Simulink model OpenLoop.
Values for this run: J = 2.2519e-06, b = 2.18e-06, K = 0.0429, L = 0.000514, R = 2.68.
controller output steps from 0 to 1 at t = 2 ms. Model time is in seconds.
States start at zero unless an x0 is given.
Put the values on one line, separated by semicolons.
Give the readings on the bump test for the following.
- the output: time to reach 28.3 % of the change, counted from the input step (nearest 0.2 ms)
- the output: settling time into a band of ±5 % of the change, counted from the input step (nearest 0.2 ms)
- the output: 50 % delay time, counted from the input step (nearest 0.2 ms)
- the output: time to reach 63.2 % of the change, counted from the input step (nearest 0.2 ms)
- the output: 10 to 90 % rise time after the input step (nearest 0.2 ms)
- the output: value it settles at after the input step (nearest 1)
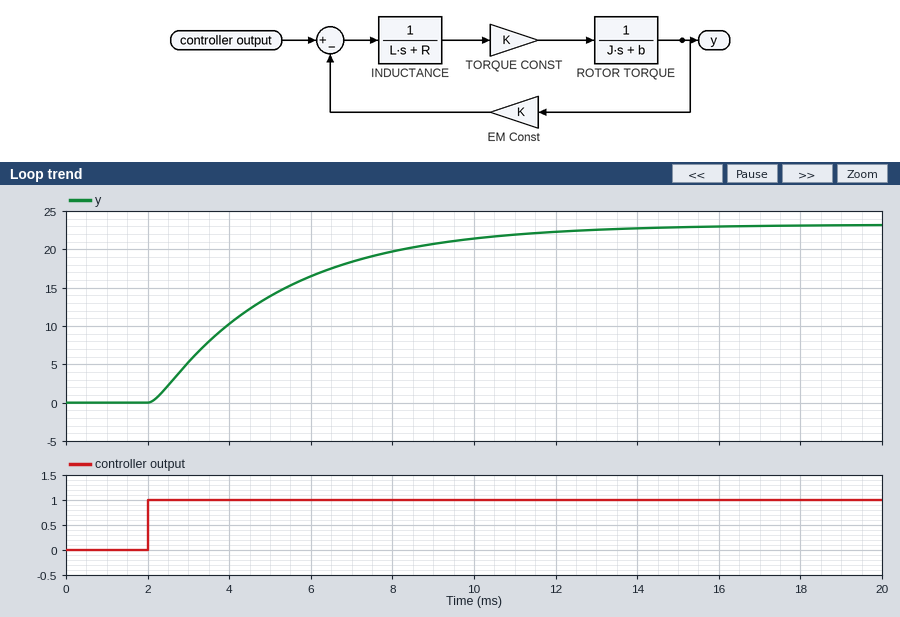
1.2 ms; 9.4 ms; 2.4 ms; 3.2 ms; 6.8 ms; 23
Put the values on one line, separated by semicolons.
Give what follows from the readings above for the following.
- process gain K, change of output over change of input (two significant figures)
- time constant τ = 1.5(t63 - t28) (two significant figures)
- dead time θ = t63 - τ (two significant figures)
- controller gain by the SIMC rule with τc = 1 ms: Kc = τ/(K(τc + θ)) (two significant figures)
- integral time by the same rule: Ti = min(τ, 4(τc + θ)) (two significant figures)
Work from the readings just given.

23; 3.0 ms; 0.20 ms; 0.11; 3.0 ms
